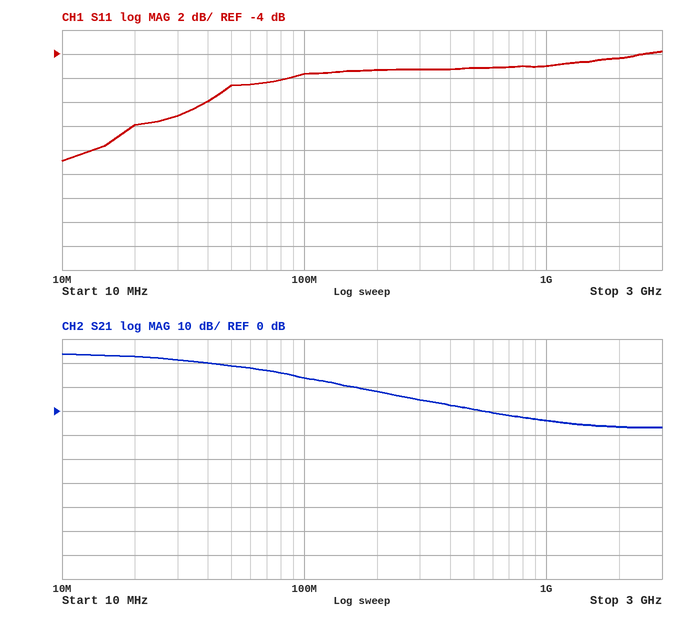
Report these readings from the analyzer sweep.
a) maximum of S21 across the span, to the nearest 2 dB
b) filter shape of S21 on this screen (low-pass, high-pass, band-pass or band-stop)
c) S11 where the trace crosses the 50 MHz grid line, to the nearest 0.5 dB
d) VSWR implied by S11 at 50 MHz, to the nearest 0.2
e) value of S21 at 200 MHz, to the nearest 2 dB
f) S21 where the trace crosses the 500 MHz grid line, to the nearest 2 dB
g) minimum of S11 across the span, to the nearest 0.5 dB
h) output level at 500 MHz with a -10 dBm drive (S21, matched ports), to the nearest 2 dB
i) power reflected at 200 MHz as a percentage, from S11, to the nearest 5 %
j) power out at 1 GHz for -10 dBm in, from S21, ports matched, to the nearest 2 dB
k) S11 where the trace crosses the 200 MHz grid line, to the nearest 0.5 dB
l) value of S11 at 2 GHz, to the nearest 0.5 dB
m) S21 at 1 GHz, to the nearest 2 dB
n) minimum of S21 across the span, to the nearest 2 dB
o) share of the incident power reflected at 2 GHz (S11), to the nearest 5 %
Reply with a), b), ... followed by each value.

a) 24 dB
b) low-pass
c) -6.5 dB
d) 2.8
e) 8 dB
f) 0 dB
g) -13.0 dB
h) -10 dBm
i) 30 %
j) -14 dBm
k) -5.5 dB
l) -4.5 dB
m) -4 dB
n) -6 dB
o) 35 %
